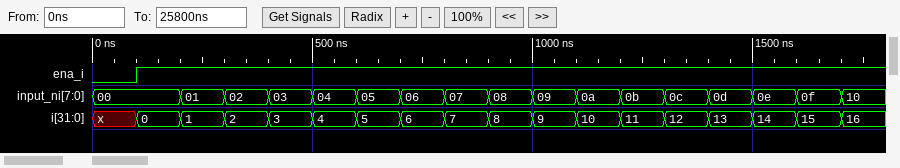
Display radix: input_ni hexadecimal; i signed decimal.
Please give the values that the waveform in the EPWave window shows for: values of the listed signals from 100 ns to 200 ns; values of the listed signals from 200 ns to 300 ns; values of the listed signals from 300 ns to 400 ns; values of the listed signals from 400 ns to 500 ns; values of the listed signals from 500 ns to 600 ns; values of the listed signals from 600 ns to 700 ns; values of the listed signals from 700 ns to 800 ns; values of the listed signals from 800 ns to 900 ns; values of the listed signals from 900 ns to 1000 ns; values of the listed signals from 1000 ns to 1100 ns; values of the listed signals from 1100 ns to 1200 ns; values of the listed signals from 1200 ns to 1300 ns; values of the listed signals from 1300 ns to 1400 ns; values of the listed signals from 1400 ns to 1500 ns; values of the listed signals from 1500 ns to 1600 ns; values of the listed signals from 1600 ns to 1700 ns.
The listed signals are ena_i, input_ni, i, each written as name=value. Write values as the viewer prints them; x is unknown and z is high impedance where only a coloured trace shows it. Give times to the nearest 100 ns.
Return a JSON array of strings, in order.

["ena_i=1, input_ni=00, i=0", "ena_i=1, input_ni=01, i=1", "ena_i=1, input_ni=02, i=2", "ena_i=1, input_ni=03, i=3", "ena_i=1, input_ni=04, i=4", "ena_i=1, input_ni=05, i=5", "ena_i=1, input_ni=06, i=6", "ena_i=1, input_ni=07, i=7", "ena_i=1, input_ni=08, i=8", "ena_i=1, input_ni=09, i=9", "ena_i=1, input_ni=0a, i=10", "ena_i=1, input_ni=0b, i=11", "ena_i=1, input_ni=0c, i=12", "ena_i=1, input_ni=0d, i=13", "ena_i=1, input_ni=0e, i=14", "ena_i=1, input_ni=0f, i=15"]
